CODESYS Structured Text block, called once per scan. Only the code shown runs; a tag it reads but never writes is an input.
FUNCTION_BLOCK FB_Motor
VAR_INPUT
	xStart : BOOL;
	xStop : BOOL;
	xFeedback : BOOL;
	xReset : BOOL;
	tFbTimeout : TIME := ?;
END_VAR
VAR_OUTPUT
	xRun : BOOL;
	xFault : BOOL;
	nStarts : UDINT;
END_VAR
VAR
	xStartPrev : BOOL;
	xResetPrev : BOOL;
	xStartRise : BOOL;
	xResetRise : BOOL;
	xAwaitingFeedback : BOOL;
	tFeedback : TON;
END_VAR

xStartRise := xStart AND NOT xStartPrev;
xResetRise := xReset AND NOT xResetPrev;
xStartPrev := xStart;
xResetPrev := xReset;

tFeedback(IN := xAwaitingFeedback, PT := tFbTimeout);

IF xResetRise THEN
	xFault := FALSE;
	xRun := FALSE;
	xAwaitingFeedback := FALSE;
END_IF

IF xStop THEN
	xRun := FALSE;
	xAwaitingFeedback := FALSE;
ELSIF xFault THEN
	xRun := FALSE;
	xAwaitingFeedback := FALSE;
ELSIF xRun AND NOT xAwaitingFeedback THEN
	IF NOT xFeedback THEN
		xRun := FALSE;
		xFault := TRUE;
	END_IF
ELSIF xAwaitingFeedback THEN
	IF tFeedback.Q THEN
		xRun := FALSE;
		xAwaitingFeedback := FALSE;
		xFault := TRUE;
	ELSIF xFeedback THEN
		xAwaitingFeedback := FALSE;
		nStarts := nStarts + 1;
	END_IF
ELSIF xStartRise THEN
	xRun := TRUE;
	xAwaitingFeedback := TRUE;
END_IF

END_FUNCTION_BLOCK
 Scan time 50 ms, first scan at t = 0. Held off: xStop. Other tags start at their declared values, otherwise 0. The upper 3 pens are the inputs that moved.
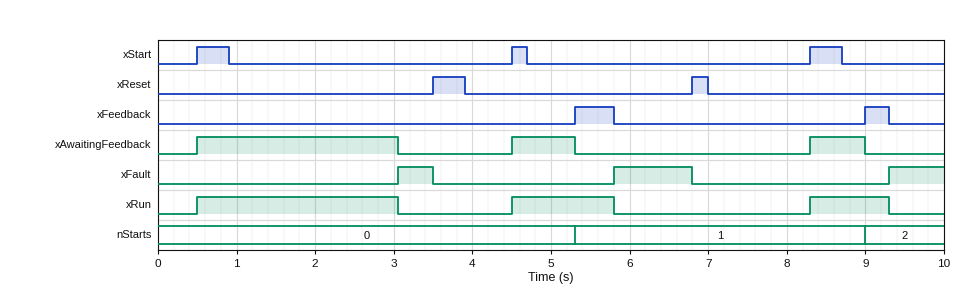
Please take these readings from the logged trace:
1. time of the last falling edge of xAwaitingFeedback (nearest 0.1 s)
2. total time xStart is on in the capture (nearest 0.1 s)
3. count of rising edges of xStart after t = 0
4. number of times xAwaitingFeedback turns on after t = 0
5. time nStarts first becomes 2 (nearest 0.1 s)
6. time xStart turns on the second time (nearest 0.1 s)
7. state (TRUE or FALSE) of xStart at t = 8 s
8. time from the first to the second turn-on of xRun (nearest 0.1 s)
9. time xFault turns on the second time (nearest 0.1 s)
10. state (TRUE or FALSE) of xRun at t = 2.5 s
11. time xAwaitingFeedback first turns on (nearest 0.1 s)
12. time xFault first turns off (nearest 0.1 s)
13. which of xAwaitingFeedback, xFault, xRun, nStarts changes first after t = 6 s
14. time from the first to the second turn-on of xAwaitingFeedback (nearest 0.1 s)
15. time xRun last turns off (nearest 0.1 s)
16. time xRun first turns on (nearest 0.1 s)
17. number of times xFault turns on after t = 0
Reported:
9.0 s
1.0 s
3
3
9.0 s
4.5 s
FALSE
4.0 s
5.8 s
TRUE
0.5 s
3.5 s
xFault
4.0 s
9.3 s
0.5 s
3
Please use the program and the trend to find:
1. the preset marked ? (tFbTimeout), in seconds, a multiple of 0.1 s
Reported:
2.5 s
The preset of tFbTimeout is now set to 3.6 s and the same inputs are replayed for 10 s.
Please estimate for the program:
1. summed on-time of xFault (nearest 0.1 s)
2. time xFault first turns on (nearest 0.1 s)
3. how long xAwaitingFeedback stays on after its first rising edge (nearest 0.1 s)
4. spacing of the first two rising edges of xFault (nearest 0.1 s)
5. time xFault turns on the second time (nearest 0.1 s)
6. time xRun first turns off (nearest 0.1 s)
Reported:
1.7 s
5.8 s
3.0 s
3.5 s
9.3 s
3.5 s
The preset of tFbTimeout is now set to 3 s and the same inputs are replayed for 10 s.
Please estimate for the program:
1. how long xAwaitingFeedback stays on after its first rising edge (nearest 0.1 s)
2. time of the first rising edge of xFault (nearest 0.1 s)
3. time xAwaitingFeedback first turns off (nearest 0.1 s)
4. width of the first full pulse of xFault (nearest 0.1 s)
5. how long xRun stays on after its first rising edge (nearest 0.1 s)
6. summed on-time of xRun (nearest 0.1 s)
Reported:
3.0 s
5.8 s
3.5 s
1.0 s
3.0 s
5.3 s
